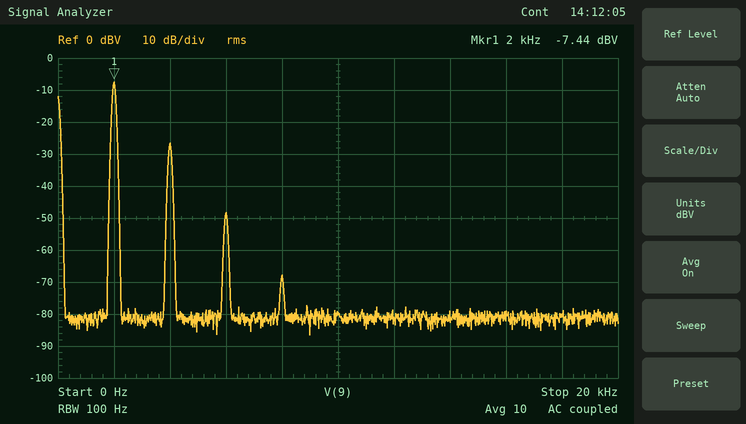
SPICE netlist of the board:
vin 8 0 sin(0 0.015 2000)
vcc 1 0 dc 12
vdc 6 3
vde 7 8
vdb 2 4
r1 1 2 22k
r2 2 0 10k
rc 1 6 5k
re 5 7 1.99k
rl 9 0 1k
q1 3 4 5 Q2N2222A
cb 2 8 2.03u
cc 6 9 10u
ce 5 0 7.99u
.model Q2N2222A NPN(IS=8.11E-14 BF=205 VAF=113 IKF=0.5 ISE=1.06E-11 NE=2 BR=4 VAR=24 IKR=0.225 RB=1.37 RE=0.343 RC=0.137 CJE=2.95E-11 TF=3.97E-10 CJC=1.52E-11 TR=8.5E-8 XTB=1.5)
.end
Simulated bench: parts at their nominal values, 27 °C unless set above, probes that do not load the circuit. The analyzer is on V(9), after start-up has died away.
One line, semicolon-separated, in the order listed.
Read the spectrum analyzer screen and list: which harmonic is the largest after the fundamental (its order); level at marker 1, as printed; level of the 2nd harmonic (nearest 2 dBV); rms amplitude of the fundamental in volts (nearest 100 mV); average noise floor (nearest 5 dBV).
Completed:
2; -7.44 dBV; -26 dBV; 400 mV; -80 dBV
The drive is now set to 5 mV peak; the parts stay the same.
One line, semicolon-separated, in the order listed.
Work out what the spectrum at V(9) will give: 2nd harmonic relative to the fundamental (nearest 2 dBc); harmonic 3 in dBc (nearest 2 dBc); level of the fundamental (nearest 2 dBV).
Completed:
-28 dBc; -60 dBc; -16 dBV
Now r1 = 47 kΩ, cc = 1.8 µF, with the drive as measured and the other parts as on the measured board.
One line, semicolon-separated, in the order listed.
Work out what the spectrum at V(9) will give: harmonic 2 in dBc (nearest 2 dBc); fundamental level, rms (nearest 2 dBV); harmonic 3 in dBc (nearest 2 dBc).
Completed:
-18 dBc; -12 dBV; -38 dBc
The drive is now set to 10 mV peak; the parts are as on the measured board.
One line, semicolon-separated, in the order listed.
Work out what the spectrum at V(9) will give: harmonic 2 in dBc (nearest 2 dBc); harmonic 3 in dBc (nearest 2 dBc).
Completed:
-22 dBc; -48 dBc
